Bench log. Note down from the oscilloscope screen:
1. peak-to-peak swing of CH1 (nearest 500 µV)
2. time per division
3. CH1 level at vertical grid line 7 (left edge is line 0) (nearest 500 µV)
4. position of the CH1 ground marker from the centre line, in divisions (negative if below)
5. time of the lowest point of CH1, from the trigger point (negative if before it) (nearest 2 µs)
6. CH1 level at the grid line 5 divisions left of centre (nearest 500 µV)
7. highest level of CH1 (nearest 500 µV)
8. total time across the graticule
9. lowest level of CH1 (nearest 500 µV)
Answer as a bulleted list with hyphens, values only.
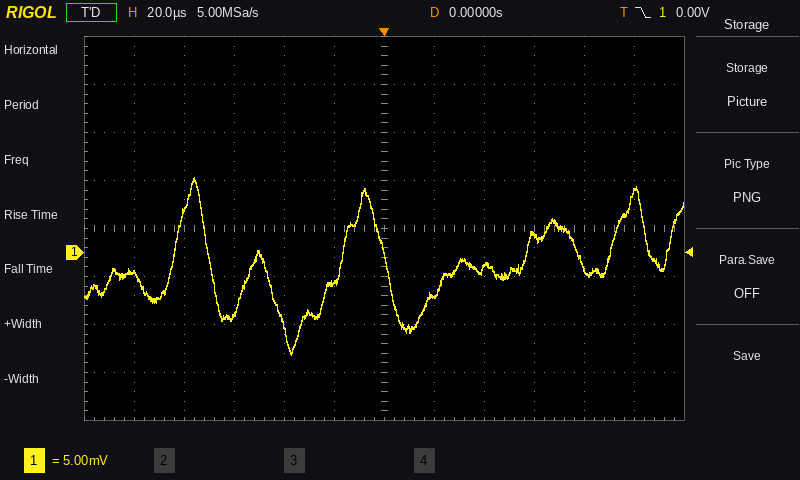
- 18.5 mV
- 20 µs
- -4.5 mV
- -0.5 div
- -38 µs
- -2.0 mV
- 8.0 mV
- 240 µs
- -10.5 mV
